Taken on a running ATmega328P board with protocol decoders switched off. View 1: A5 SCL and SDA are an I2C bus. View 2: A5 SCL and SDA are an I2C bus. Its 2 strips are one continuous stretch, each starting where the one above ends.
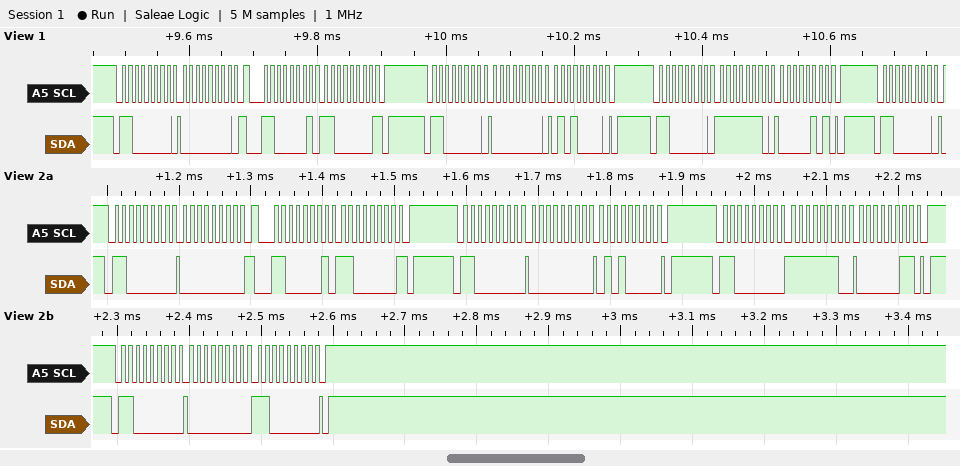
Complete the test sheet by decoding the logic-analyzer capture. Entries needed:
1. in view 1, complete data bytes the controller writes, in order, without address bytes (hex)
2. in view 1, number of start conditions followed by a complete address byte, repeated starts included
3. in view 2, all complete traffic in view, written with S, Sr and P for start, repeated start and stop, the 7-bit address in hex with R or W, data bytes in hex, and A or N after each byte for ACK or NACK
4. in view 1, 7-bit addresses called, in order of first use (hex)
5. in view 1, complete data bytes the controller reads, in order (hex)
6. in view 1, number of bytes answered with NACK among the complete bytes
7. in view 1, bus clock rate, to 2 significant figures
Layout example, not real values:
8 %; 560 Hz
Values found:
00 00 50 FE 05; 5; S 60W A 00 A Sr 60R A C0 N P S 60W A 00 A 50 A P S 60W A FE A 03 A P S 60W A 00 A C0 A P; 0x60; C0; 1; 100 kHz
